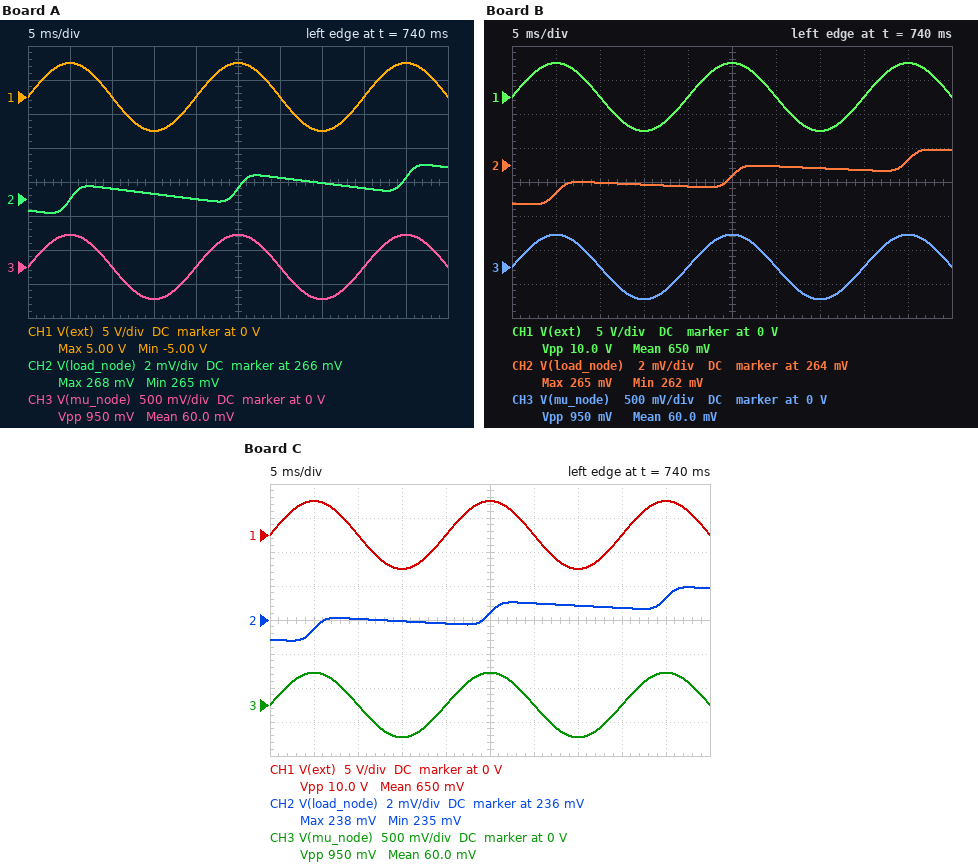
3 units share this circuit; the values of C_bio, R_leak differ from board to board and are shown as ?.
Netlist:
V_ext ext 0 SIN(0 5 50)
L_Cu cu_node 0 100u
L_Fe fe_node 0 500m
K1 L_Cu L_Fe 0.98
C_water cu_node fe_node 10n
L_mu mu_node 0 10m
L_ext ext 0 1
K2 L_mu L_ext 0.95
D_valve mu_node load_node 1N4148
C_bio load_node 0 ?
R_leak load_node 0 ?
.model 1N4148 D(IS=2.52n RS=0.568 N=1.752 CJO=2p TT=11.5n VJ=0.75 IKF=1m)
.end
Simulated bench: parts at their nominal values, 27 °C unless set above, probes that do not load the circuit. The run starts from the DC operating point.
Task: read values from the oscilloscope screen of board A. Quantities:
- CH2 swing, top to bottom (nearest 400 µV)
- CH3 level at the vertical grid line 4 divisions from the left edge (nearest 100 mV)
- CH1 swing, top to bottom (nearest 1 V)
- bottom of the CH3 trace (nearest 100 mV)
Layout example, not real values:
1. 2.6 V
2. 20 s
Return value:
1. 2.8 mV
2. 0 V
3. 10 V
4. -500 mV
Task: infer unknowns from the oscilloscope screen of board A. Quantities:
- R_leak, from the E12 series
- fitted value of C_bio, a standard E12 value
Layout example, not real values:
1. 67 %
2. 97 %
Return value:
1. 15 MΩ
2. 330 nF
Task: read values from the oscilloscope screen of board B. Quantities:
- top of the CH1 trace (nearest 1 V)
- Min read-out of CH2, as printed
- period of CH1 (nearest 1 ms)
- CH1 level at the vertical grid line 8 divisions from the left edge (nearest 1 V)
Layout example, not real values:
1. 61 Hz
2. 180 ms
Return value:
1. 5 V
2. 262 mV
3. 20 ms
4. 0 V
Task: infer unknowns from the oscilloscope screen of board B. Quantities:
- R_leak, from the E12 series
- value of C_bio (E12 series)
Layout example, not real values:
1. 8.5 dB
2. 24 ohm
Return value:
1. 33 MΩ
2. 470 nF
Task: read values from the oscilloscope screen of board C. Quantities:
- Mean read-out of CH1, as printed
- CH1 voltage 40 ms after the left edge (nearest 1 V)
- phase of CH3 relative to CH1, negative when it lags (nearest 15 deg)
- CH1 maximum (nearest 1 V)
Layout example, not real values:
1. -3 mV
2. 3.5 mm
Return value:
1. 650 mV
2. 0 V
3. 0 deg
4. 5 V
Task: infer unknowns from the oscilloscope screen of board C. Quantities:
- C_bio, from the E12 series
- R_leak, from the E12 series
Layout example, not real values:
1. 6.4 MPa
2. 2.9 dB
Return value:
1. 820 nF
2. 12 MΩ
